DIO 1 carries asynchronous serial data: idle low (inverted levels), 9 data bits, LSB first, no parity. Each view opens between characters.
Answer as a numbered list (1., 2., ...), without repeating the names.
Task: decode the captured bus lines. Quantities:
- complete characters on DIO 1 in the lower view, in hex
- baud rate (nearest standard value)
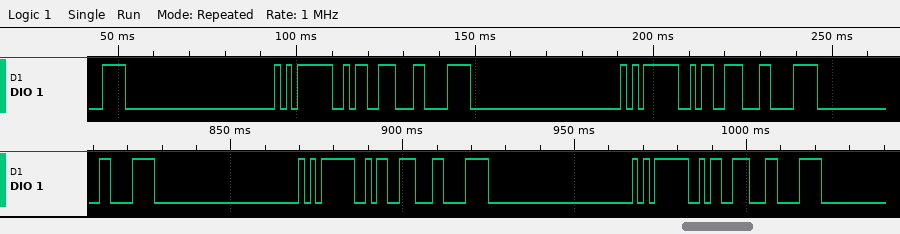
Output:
1. 1E, 05, 119, 1E, 05, 119, 1E
2. 600 baud
